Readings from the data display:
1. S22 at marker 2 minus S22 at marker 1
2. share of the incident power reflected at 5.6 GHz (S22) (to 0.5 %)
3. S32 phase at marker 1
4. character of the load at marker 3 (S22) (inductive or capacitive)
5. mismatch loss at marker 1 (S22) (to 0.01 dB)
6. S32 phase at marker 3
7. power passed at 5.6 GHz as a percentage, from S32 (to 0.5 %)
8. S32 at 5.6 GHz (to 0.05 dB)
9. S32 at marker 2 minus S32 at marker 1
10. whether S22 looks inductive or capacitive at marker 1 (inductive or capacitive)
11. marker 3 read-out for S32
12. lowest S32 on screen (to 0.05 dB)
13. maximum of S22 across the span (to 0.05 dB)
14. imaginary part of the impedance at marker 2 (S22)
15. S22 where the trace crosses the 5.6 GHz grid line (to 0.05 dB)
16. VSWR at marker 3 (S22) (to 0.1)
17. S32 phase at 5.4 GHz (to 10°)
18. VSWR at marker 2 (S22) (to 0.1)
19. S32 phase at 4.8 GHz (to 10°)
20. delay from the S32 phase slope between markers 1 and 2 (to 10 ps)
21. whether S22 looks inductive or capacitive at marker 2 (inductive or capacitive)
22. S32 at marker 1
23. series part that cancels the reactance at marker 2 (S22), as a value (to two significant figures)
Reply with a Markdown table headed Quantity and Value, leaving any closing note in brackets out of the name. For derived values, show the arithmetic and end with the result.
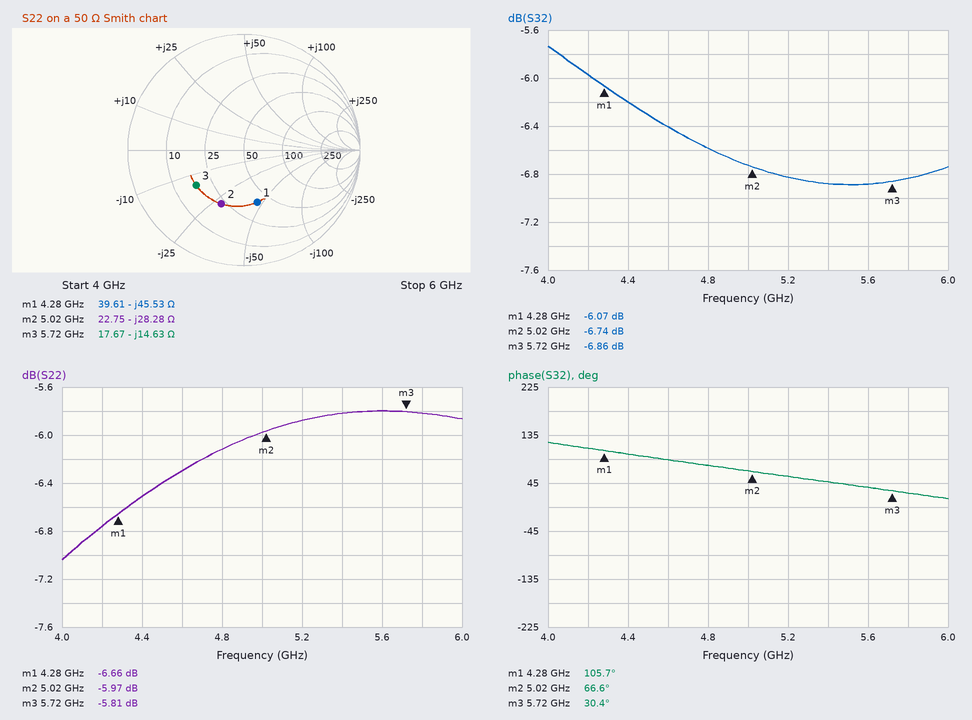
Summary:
| Quantity | Value |
|---|---|
| S22 at marker 2 minus S22 at marker 1 | -5.97 − (-6.66) = 0.69 dB |
| share of the incident power reflected at 5.6 GHz (S22) | 10^(-5.8/10) ≈ 26.3 %, so 26.5 % to the nearest 0.5 % |
| S32 phase at marker 1 | 105.7° |
| character of the load at marker 3 (S22) | capacitive |
| mismatch loss at marker 1 (S22) | −10 log10(1 − 10^(-6.66/10)) ≈ 1.06 dB |
| S32 phase at marker 3 | 30.4° |
| power passed at 5.6 GHz as a percentage, from S32 | 10^(-6.9/10) ≈ 20.4 %, so 20.5 % to the nearest 0.5 % |
| S32 at 5.6 GHz | -6.90 dB |
| S32 at marker 2 minus S32 at marker 1 | -6.74 − (-6.07) = -0.67 dB |
| whether S22 looks inductive or capacitive at marker 1 | capacitive |
| marker 3 read-out for S32 | -6.86 dB |
| lowest S32 on screen | -6.90 dB |
| maximum of S22 across the span | -5.80 dB |
| imaginary part of the impedance at marker 2 | -28.28 Ω |
| S22 where the trace crosses the 5.6 GHz grid line | -5.80 dB |
| VSWR at marker 3 (S22) | (1 + 0.5123)/(1 − 0.5123) ≈ 3.1 |
| S32 phase at 5.4 GHz | 50° |
| VSWR at marker 2 (S22) | 3.0 |
| S32 phase at 4.8 GHz | 80° |
| delay from the S32 phase slope between markers 1 and 2 | −(66.6° − (105.7°))/(360° × 740 MHz) ≈ 147 ps, so 150 ps to the nearest 10 ps |
| whether S22 looks inductive or capacitive at marker 2 | capacitive |
| S32 at marker 1 | -6.07 dB |
| series part that cancels the reactance at marker 2 (S22), as a value | L = 28.28 Ω/(2π × 5.02 GHz) ≈ 897 pH, so 900 pH to two significant figures |
